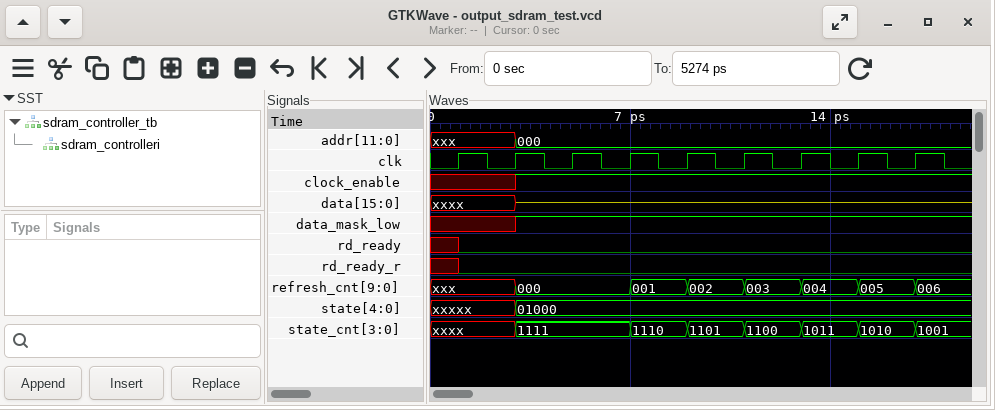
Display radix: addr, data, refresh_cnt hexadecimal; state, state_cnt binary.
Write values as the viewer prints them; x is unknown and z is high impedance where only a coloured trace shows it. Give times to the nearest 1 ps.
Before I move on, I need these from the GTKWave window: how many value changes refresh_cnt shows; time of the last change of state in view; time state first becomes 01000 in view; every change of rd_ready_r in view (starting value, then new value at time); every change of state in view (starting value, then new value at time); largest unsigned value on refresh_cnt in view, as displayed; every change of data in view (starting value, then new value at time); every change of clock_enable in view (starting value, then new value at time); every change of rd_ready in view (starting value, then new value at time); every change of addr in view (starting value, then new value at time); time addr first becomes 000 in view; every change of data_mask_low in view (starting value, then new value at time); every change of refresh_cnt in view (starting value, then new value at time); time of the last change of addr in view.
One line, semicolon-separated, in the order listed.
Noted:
7; 3 ps; 3 ps; x, 0 at 1 ps; xxxxx, 01000 at 3 ps; 006; xxxx, z at 3 ps; x, 1 at 3 ps; x, 0 at 1 ps; xxx, 000 at 3 ps; 3 ps; x, 1 at 3 ps; xxx, 000 at 3 ps, 001 at 7 ps, 002 at 9 ps, 003 at 11 ps, 004 at 13 ps, 005 at 15 ps, 006 at 17 ps; 3 ps
